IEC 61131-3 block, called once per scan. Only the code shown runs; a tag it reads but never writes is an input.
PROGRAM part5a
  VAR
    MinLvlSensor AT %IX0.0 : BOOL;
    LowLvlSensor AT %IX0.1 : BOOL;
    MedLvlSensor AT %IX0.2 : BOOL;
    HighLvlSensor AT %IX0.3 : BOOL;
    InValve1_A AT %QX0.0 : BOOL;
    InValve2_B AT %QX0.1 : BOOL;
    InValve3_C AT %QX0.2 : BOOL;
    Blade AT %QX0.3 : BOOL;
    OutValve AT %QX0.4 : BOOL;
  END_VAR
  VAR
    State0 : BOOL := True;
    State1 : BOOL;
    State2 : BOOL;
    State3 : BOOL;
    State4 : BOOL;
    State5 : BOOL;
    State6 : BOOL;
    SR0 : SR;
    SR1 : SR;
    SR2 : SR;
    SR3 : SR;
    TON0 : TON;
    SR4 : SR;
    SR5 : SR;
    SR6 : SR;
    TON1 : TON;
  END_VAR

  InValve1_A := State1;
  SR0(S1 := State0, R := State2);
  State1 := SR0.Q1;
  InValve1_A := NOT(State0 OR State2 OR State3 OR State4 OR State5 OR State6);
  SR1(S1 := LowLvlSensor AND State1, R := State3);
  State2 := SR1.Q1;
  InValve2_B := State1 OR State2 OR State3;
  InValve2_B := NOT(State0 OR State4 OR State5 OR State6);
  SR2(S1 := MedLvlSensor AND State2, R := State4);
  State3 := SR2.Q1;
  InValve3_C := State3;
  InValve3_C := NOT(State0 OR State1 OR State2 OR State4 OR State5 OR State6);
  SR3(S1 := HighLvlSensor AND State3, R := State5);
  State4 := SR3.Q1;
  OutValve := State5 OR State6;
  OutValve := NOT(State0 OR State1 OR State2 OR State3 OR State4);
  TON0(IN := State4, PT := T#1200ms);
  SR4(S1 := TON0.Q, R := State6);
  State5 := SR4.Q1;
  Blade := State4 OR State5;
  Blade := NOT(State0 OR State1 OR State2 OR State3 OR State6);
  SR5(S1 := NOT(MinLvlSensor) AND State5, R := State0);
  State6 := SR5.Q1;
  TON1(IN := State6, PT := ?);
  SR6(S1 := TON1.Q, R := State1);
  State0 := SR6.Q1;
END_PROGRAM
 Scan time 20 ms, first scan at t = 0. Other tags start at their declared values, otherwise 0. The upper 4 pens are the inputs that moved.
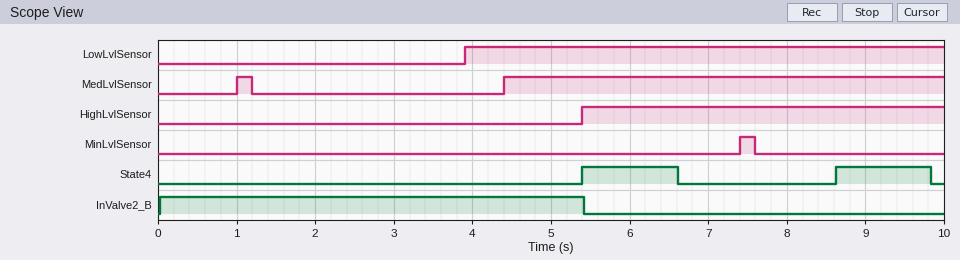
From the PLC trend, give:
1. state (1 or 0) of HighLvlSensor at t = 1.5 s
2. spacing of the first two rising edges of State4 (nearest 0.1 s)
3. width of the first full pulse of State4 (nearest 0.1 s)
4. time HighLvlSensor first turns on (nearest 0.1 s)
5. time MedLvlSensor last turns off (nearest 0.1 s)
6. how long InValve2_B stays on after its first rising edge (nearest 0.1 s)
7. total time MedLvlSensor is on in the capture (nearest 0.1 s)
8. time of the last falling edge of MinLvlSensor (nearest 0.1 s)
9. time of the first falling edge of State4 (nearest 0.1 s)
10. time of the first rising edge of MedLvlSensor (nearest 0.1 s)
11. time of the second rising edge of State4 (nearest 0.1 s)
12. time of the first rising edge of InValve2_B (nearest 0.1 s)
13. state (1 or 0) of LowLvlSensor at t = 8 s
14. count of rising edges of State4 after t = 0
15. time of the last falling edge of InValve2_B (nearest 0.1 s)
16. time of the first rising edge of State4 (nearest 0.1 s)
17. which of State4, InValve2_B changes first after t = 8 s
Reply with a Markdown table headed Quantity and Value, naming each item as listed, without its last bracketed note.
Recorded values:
| Quantity | Value |
|---|---|
| state (1 or 0) of HighLvlSensor at t = 1.5 s | 0 |
| spacing of the first two rising edges of State4 | 3.2 s |
| width of the first full pulse of State4 | 1.2 s |
| time HighLvlSensor first turns on | 5.4 s |
| time MedLvlSensor last turns off | 1.2 s |
| how long InValve2_B stays on after its first rising edge | 5.4 s |
| total time MedLvlSensor is on in the capture | 5.8 s |
| time of the last falling edge of MinLvlSensor | 7.6 s |
| time of the first falling edge of State4 | 6.6 s |
| time of the first rising edge of MedLvlSensor | 1.0 s |
| time of the second rising edge of State4 | 8.6 s |
| time of the first rising edge of InValve2_B | 0.0 s |
| state (1 or 0) of LowLvlSensor at t = 8 s | 1 |
| count of rising edges of State4 after t = 0 | 2 |
| time of the last falling edge of InValve2_B | 5.4 s |
| time of the first rising edge of State4 | 5.4 s |
| which of State4, InValve2_B changes first after t = 8 s | State4 |
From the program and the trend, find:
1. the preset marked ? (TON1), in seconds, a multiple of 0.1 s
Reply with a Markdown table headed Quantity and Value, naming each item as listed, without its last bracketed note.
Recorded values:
| Quantity | Value |
|---|---|
| the preset marked ? (TON1), in seconds, a multiple of 0.1 s | 2.0 s |
